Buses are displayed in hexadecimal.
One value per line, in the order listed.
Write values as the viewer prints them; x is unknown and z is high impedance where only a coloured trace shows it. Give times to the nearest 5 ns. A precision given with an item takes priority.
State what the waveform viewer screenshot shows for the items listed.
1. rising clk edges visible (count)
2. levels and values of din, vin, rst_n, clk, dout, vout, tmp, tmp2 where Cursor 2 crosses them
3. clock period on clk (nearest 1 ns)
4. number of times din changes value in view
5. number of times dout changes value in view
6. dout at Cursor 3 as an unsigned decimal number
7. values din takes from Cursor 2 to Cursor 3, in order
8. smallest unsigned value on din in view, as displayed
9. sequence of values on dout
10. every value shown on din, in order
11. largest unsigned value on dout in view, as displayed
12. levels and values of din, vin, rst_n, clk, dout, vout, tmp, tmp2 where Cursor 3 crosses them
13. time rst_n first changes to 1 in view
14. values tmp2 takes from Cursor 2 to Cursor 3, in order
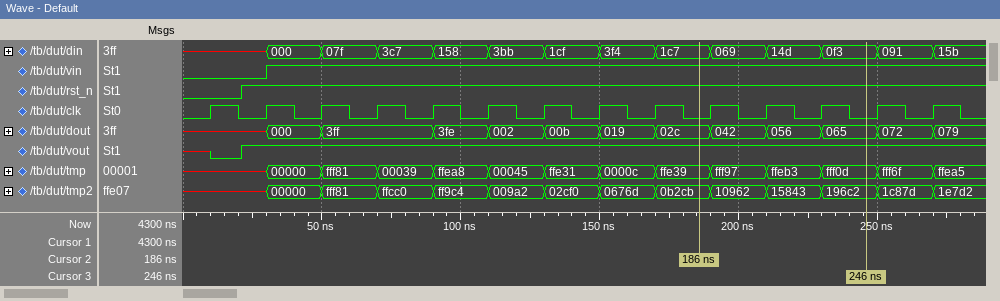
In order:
14
din=1c7, vin=1, rst_n=1, clk=0, dout=02c, vout=1, tmp=ffe39, tmp2=0b2cb
20 ns
13
12
101
1c7, 069, 14d, 0f3
000
x, 000, 3ff, 3fe, 002, 00b, 019, 02c, 042, 056, 065, 072, 079
x, 000, 07f, 3c7, 158, 3bb, 1cf, 3f4, 1c7, 069, 14d, 0f3, 091, 15b
3ff
din=0f3, vin=1, rst_n=1, clk=0, dout=065, vout=1, tmp=fff0d, tmp2=196c2
20 ns
0b2cb, 10962, 15843, 196c2
